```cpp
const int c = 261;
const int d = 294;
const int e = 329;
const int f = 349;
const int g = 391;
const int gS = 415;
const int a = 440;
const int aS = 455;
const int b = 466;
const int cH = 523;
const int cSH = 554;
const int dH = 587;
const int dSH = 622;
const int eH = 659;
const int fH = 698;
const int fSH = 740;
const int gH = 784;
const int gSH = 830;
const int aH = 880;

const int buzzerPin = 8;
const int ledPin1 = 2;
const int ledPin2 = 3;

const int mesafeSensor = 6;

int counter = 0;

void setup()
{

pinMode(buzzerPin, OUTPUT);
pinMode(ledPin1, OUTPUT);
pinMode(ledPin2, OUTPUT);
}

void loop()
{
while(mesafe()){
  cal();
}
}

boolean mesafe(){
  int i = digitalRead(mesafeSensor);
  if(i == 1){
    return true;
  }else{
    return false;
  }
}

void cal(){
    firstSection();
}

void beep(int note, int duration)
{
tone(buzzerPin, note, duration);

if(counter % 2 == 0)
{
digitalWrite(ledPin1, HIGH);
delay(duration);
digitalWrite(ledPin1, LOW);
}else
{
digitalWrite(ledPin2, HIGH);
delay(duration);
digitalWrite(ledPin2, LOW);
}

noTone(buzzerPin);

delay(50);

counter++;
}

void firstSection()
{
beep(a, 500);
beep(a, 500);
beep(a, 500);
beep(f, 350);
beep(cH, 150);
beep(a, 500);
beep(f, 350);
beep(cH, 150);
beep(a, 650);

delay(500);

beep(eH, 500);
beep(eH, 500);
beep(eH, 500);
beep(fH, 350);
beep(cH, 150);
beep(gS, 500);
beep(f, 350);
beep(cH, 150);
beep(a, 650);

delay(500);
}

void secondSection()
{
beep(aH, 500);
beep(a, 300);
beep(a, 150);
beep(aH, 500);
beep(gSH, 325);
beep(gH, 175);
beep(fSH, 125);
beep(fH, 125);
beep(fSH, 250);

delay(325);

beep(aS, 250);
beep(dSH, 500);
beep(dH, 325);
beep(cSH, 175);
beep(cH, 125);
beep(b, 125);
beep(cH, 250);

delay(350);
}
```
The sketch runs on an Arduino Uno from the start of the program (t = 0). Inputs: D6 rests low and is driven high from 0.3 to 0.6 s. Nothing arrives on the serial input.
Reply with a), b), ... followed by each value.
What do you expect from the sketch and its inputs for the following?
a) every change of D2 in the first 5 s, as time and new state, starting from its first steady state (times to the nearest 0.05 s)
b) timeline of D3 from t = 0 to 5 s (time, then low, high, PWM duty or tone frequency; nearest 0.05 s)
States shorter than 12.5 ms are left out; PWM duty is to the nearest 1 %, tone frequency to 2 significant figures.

a) 0 s low; 0.3 s high; 0.8 s low; 1.4 s high; 1.9 s low; 2.35 s high; 2.5 s low; 3.1 s high; 3.45 s low; 3.7 s high; 4.35 s low
b) 0 s low; 0.85 s high; 1.35 s low; 1.95 s high; 2.3 s low; 2.55 s high; 3.05 s low; 3.5 s high; 3.65 s low; 4.9 s high
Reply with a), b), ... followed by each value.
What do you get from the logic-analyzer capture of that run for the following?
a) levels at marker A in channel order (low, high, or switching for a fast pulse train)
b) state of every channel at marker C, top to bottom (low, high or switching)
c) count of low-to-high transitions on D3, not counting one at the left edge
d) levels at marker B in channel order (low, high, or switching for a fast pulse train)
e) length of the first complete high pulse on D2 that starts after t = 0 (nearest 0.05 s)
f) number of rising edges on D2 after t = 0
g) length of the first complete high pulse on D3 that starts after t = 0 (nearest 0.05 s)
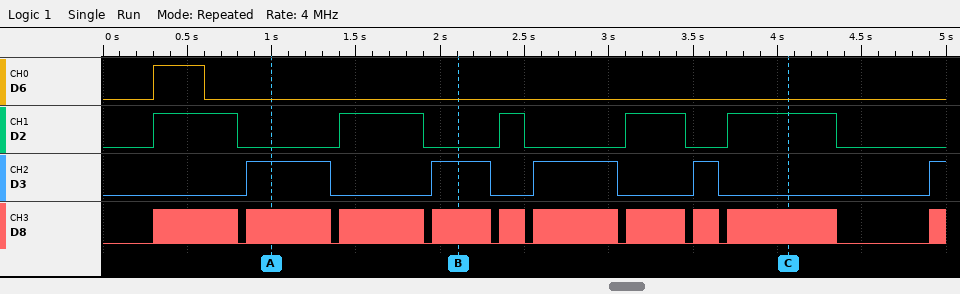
a) D6 low, D2 low, D3 high, D8 switching
b) D6 low, D2 high, D3 low, D8 switching
c) 5
d) D6 low, D2 low, D3 high, D8 switching
e) 0.50 s
f) 5
g) 0.50 s
